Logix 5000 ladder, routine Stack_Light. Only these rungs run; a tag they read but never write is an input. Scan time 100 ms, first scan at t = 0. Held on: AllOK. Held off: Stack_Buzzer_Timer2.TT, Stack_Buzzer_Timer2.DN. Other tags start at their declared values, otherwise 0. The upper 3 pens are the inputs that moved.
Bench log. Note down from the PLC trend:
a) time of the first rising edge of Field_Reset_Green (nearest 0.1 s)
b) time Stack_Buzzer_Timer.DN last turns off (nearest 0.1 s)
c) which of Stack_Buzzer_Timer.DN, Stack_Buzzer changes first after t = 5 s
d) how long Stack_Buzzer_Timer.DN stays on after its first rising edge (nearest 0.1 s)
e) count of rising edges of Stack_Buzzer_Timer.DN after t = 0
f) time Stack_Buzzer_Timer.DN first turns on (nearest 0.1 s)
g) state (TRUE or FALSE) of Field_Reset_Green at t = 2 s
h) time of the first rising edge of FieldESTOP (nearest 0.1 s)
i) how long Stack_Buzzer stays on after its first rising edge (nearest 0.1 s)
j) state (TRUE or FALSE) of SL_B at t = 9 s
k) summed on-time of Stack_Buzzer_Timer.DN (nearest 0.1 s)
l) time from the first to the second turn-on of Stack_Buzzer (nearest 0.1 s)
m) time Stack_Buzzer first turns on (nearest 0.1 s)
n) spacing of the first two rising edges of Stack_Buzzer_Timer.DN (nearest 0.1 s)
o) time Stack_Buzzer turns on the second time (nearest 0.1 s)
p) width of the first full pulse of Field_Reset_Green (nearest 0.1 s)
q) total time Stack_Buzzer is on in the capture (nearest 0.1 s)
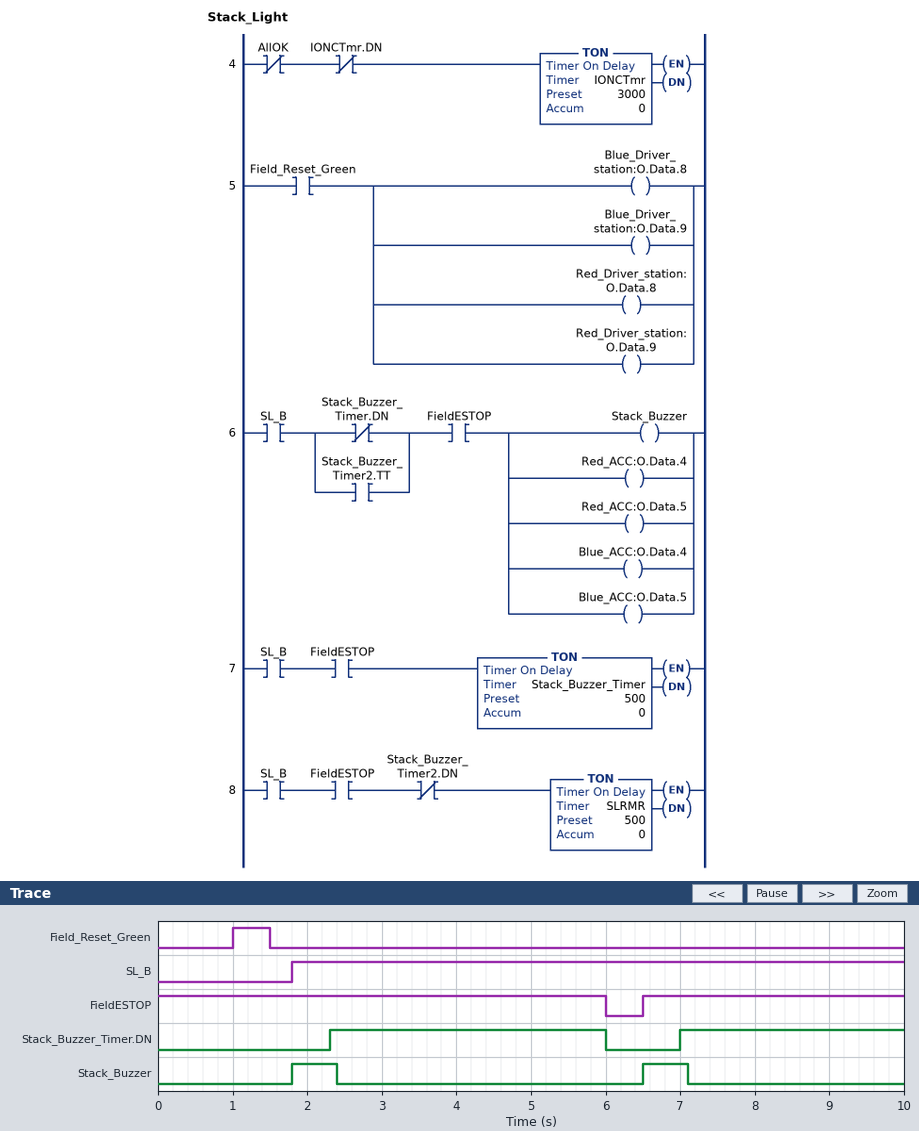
1.0 s
6.0 s
Stack_Buzzer_Timer.DN
3.7 s
2
2.3 s
FALSE
6.5 s
0.6 s
TRUE
6.7 s
4.7 s
1.8 s
4.7 s
6.5 s
0.5 s
1.2 s
